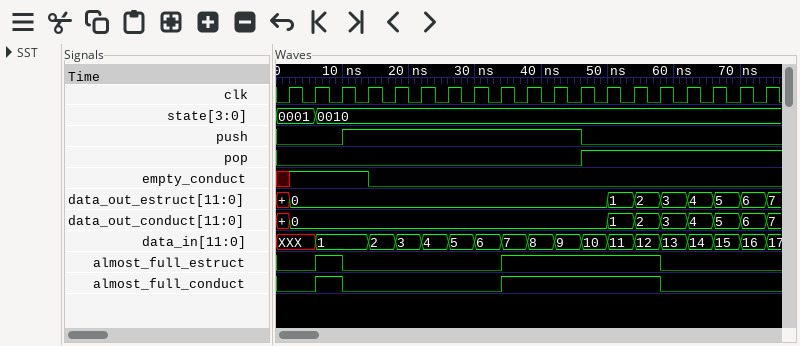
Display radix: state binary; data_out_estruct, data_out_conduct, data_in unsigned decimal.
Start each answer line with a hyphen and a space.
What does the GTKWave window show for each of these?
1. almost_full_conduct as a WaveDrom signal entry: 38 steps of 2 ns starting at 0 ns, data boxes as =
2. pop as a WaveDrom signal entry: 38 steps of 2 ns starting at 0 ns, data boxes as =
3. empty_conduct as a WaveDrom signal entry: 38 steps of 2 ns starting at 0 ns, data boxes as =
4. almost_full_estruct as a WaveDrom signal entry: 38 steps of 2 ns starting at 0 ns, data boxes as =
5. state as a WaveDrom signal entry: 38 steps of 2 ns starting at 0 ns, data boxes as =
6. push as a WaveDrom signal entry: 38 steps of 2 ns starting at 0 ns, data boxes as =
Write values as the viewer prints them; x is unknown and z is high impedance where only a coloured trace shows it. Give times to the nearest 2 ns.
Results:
- {name: 'almost_full_conduct', wave: '0..1.0...........1...........0........'}
- {name: 'pop', wave: '0......................1..............'}
- {name: 'empty_conduct', wave: 'x1.....0..............................'}
- {name: 'almost_full_estruct', wave: '0..1.0...........1...........0........'}
- {name: 'state', wave: '=..=..................................', data: '0001 0010'}
- {name: 'push', wave: '0....1.................0..............'}
